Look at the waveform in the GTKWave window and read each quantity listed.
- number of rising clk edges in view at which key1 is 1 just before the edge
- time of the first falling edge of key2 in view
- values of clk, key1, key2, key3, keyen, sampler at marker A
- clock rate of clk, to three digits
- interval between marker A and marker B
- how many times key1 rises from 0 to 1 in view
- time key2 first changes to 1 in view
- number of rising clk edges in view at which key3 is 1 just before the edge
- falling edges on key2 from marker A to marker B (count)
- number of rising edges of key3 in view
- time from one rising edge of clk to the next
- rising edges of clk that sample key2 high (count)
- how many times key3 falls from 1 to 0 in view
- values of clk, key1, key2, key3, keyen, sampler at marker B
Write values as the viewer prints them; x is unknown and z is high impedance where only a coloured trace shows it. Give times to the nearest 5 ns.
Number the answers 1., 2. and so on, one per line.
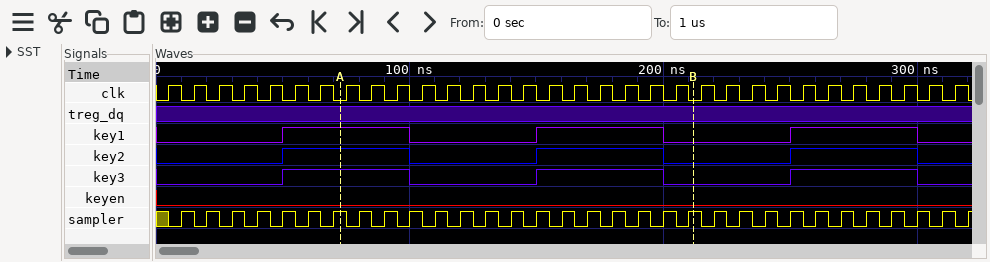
1. 15
2. 100 ns
3. clk=0, key1=1, key2=1, key3=1, keyen=0, sampler=1
4. 100 MHz
5. 140 ns
6. 3
7. 50 ns
8. 15
9. 2
10. 3
11. 10 ns
12. 15
13. 3
14. clk=0, key1=0, key2=0, key3=0, keyen=0, sampler=1
